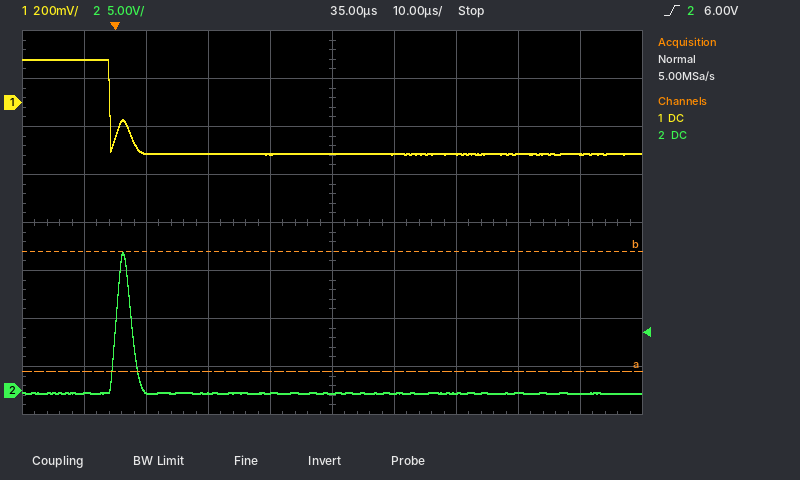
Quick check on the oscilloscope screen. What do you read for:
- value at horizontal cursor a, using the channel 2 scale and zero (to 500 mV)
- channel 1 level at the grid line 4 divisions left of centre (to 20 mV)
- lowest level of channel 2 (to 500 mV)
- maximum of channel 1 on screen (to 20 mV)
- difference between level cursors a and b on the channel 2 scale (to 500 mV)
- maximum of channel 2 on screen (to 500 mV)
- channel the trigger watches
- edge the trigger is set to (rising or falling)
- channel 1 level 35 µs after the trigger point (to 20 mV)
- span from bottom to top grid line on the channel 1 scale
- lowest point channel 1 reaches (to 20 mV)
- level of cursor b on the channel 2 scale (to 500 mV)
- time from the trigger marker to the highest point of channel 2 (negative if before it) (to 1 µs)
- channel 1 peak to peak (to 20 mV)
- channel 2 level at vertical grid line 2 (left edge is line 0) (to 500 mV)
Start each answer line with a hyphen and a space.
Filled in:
- 2.0 V
- 180 mV
- -500 mV
- 180 mV
- 12.5 V
- 14.5 V
- channel 2
- rising
- -220 mV
- 1.6 V
- -220 mV
- 14.5 V
- +1 µs
- 400 mV
- 0.0 V
